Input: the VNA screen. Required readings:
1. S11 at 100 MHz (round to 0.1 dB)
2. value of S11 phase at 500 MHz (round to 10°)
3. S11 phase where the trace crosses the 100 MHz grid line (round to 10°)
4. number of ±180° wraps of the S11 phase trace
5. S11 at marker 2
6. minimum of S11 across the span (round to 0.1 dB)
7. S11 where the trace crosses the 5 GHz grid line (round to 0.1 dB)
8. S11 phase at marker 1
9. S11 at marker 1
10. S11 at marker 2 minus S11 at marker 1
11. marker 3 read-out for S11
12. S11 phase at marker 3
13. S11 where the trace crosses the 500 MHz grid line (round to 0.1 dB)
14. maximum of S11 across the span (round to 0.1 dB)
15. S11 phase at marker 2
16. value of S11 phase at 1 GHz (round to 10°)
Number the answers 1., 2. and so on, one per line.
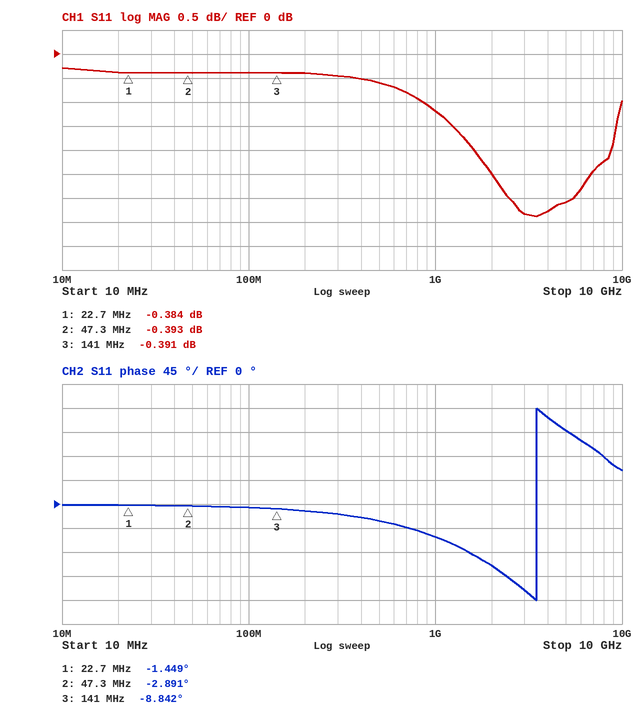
1. -0.4 dB
2. -30°
3. -10°
4. 1
5. -0.393 dB
6. -3.4 dB
7. -3.1 dB
8. -1.449°
9. -0.384 dB
10. -0.009 dB
11. -0.391 dB
12. -8.842°
13. -0.6 dB
14. -0.3 dB
15. -2.891°
16. -60°
